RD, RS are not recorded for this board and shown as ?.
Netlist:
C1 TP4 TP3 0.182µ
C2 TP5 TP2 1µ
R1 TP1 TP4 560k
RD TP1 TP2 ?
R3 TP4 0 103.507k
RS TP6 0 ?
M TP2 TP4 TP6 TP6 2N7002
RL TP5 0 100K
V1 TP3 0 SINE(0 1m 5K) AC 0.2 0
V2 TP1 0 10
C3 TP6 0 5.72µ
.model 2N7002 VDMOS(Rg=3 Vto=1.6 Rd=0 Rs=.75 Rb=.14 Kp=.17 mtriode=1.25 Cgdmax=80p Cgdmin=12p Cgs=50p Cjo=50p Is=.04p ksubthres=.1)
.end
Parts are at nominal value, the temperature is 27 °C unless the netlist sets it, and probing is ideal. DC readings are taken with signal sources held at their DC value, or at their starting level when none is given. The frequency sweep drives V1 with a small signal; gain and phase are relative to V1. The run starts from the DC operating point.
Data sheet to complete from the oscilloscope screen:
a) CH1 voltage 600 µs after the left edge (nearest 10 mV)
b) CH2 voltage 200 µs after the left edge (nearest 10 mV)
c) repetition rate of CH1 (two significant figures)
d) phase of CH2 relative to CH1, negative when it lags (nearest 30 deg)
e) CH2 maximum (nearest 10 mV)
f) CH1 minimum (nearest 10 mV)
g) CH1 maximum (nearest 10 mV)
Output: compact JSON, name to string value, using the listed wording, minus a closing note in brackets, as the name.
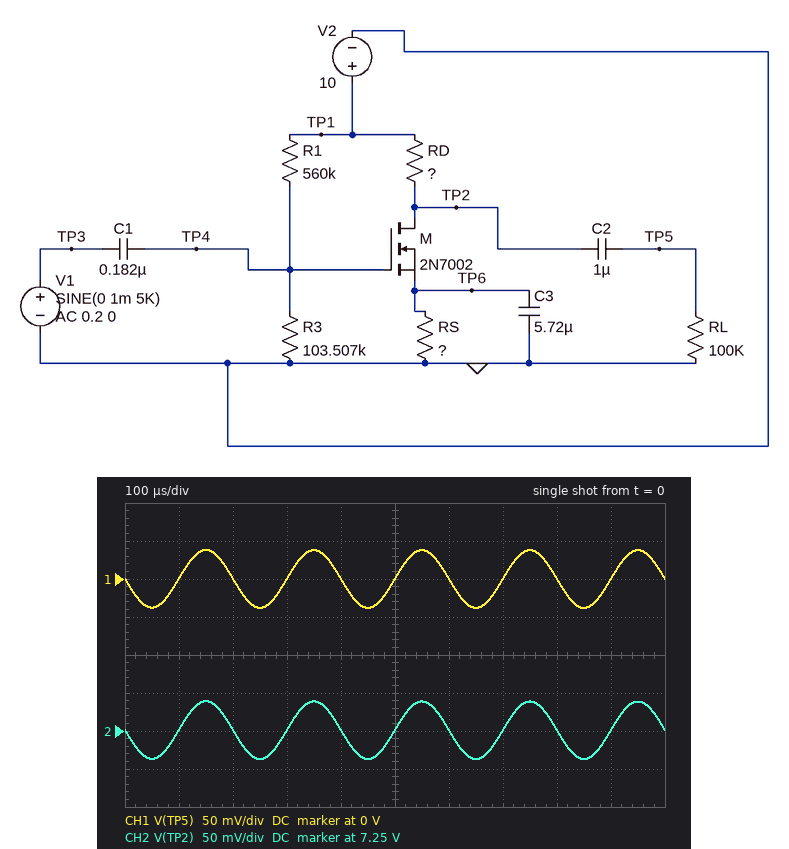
{"CH1 voltage 600 µs after the left edge": "0 V", "CH2 voltage 200 µs after the left edge": "7.25 V", "repetition rate of CH1": "5.0 kHz", "phase of CH2 relative to CH1, negative when it lags": "0 deg", "CH2 maximum": "7.29 V", "CH1 minimum": "-40 mV", "CH1 maximum": "40 mV"}
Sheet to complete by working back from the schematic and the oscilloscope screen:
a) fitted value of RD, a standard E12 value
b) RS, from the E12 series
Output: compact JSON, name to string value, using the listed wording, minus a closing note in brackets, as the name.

{"fitted value of RD, a standard E12 value": "15 kΩ", "RS, from the E12 series": "68 Ω"}
